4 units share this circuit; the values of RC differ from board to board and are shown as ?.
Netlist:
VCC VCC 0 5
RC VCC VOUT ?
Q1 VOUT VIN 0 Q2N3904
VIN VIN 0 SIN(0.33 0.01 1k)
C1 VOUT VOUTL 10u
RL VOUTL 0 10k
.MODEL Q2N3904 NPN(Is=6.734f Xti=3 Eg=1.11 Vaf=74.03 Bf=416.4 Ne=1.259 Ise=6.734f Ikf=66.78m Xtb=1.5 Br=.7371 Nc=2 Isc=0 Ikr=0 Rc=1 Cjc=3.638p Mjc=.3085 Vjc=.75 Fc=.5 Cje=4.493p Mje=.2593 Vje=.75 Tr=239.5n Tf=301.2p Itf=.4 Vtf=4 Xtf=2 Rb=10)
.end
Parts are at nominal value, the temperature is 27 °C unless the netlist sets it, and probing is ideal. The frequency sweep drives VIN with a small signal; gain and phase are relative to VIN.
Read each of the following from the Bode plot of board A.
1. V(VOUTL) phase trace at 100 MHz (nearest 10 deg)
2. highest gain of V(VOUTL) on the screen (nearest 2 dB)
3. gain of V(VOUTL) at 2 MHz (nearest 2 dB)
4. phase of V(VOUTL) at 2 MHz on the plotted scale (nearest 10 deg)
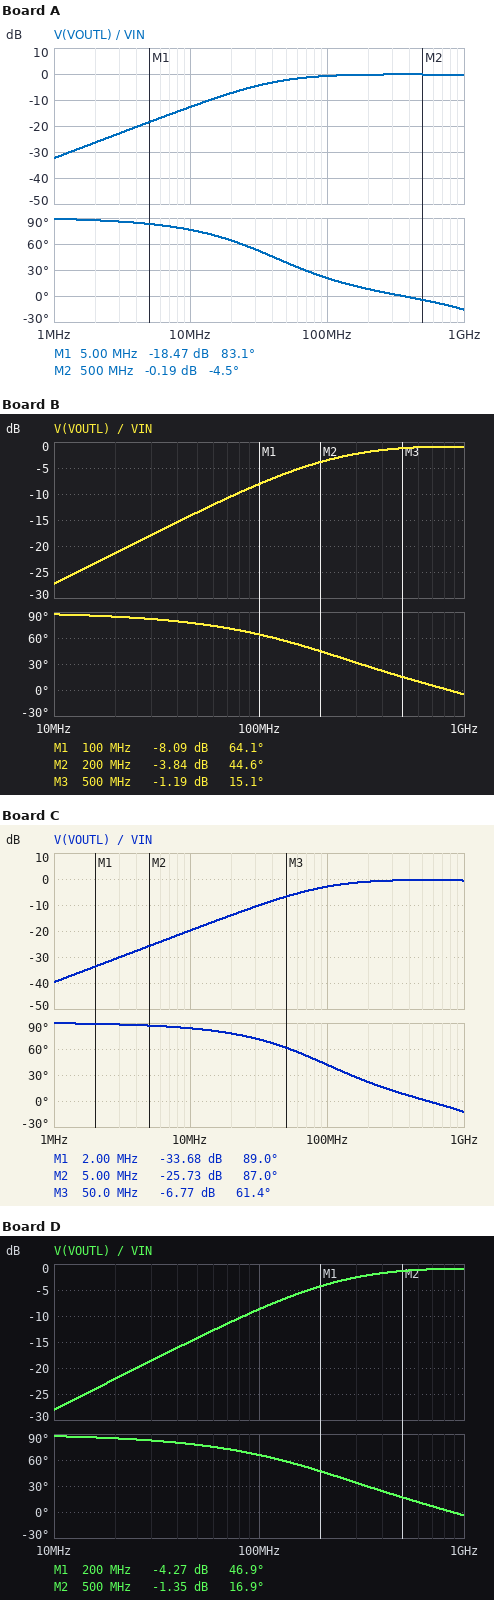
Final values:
20 deg
0 dB
-26 dB
90 deg
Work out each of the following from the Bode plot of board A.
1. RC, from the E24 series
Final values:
2.4 kΩ
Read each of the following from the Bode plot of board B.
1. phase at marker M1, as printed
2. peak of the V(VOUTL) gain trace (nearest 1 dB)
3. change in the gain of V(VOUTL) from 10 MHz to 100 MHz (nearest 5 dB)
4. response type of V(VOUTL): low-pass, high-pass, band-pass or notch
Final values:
64.1 deg
-1 dB
20 dB
high-pass
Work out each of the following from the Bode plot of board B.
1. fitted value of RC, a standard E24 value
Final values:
360 Ω
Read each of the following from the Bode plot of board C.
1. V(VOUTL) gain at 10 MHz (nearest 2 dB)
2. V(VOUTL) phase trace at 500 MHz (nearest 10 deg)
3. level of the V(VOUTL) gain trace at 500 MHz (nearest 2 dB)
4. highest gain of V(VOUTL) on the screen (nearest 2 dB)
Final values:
-20 dB
0 deg
0 dB
0 dB
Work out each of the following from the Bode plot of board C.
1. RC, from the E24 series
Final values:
910 Ω
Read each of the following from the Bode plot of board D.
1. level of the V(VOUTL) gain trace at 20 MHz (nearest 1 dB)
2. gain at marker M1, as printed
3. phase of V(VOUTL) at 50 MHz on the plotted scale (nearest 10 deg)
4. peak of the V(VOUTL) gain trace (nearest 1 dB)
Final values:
-22 dB
-4.27 dB
80 deg
-1 dB
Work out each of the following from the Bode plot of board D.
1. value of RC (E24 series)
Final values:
330 Ω
